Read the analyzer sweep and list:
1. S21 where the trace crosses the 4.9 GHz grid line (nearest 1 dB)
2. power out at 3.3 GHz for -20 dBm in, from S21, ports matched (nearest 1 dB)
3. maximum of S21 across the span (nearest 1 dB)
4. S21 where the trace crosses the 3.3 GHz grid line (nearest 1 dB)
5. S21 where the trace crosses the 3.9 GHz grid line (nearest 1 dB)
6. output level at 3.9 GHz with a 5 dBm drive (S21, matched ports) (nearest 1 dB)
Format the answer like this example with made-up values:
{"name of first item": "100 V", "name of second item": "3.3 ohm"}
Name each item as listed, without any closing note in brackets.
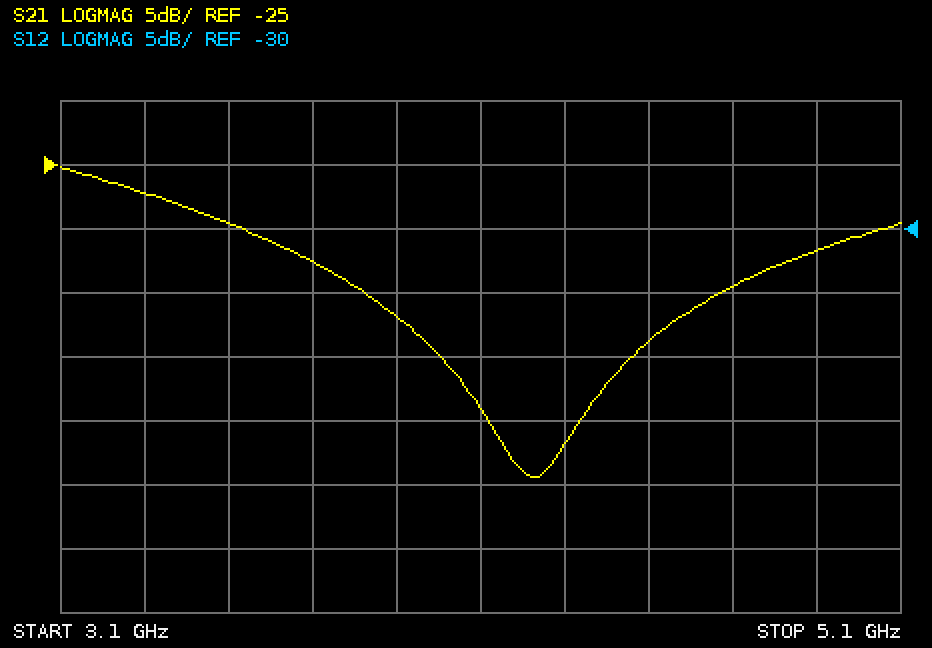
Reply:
{"S21 where the trace crosses the 4.9 GHz grid line": "-32 dB", "power out at 3.3 GHz for -20 dBm in, from S21, ports matched": "-47 dBm", "maximum of S21 across the span": "-25 dB", "S21 where the trace crosses the 3.3 GHz grid line": "-27 dB", "S21 where the trace crosses the 3.9 GHz grid line": "-37 dB", "output level at 3.9 GHz with a 5 dBm drive (S21, matched ports)": "-32 dBm"}
